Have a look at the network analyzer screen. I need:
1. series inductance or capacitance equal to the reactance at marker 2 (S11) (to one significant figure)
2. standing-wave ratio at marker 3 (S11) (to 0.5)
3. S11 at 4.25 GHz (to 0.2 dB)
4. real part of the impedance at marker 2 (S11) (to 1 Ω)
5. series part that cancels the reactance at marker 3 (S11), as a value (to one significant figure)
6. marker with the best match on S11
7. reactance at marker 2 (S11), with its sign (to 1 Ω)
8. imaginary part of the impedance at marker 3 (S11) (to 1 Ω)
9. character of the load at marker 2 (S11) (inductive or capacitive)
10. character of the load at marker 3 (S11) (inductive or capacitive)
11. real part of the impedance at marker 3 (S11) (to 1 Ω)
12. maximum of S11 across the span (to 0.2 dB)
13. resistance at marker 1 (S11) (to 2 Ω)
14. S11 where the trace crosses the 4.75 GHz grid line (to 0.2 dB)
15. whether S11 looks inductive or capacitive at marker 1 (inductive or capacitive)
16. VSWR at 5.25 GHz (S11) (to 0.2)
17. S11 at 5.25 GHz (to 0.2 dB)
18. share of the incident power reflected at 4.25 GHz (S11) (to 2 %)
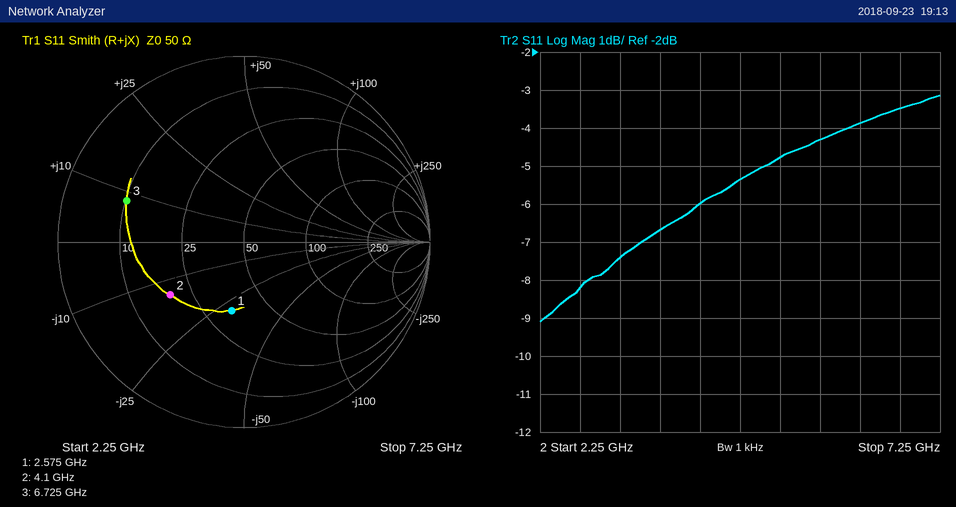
3 pF
5.0
-6.0 dB
19 Ω
3 pF
marker 1
-14 Ω
+8 Ω
capacitive
inductive
10 Ω
-3.2 dB
34 Ω
-5.4 dB
capacitive
3.8
-4.8 dB
26 %
